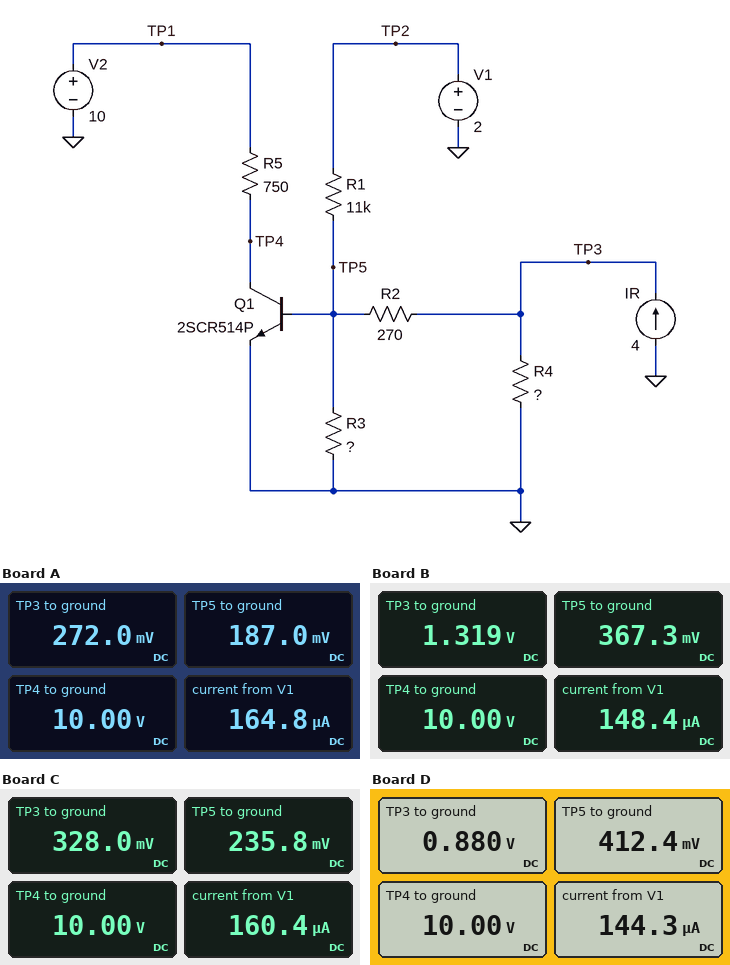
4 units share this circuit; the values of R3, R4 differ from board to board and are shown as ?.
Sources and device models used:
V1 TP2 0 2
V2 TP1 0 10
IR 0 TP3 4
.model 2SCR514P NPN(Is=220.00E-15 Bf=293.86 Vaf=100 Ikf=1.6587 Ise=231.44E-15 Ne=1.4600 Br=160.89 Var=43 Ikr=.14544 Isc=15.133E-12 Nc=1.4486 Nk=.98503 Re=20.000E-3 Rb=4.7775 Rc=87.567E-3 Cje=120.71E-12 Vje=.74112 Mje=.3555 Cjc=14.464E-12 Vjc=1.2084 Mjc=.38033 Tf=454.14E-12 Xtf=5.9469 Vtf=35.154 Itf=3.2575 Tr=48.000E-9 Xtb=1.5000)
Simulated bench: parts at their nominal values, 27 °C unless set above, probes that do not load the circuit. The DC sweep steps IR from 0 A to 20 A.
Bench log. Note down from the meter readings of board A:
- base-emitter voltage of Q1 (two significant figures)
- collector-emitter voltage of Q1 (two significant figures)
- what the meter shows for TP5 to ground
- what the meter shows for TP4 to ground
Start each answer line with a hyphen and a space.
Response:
- 190 mV
- 10 V
- 187.0 mV
- 10.00 V
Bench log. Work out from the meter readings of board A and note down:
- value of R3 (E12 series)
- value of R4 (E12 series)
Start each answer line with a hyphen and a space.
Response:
- 390 Ω
- 0.068 Ω
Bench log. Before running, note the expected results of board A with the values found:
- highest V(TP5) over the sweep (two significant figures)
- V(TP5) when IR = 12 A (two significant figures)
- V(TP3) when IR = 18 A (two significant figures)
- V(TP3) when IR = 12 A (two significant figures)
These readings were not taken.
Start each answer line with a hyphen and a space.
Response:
- 680 mV
- 500 mV
- 1.2 V
- 820 mV
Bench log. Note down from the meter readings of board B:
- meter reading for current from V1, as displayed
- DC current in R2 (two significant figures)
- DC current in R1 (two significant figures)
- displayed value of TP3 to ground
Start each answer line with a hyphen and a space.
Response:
- 148.4 µA
- 3.5 mA
- 150 µA
- 1.319 V
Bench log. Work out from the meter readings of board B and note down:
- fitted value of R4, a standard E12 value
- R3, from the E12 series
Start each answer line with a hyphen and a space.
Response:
- 0.33 Ω
- 100 Ω
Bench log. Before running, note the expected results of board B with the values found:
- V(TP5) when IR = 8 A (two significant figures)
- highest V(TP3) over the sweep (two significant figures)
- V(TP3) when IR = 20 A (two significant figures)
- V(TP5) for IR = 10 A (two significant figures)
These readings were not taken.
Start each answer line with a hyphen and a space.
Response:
- 670 mV
- 6.6 V
- 6.6 V
- 710 mV
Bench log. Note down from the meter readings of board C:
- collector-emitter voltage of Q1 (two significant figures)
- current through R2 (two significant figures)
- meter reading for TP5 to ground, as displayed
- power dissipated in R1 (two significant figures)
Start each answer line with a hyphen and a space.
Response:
- 10 V
- 340 µA
- 235.8 mV
- 280 µW
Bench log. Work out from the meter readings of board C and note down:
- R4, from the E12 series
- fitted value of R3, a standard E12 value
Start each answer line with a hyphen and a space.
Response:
- 0.082 Ω
- 470 Ω
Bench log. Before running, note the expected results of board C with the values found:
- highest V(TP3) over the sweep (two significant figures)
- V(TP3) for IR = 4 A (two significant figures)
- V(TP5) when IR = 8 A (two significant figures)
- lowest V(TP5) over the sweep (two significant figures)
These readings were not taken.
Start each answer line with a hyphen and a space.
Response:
- 1.6 V
- 330 mV
- 440 mV
- 31 mV
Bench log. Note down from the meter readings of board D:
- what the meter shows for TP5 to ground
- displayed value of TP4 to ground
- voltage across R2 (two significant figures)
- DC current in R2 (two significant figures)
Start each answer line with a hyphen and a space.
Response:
- 412.4 mV
- 10.00 V
- 470 mV
- 1.7 mA
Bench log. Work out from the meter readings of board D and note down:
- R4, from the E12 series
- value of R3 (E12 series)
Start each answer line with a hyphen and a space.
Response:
- 0.22 Ω
- 220 Ω
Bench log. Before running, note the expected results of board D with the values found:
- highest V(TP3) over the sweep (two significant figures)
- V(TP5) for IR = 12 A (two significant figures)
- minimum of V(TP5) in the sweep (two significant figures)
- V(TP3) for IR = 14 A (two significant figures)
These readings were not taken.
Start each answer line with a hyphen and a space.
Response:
- 4.4 V
- 730 mV
- 22 mV
- 3.1 V
